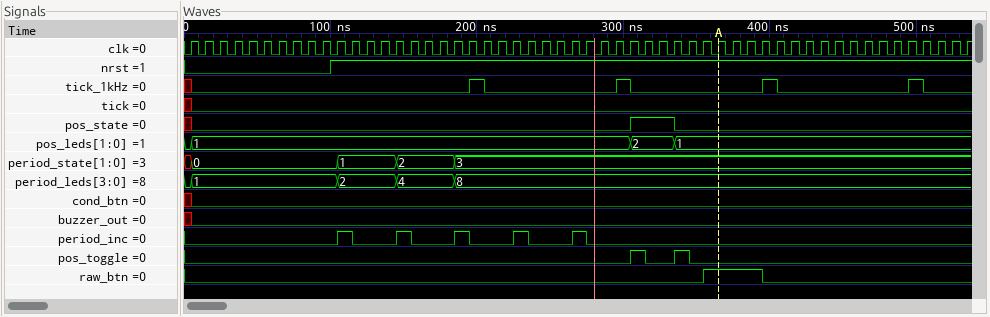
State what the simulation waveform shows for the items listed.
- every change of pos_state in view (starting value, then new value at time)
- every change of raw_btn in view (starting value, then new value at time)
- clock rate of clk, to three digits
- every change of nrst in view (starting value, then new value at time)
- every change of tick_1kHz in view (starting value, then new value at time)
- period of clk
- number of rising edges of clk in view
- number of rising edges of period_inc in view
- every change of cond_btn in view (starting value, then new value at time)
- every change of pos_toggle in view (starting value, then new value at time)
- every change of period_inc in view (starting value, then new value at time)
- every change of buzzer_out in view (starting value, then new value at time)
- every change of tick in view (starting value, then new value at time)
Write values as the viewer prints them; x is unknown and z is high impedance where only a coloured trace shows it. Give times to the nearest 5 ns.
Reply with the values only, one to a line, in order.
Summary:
x, 0 at 5 ns, 1 at 305 ns, 0 at 335 ns
0, 1 at 355 ns, 0 at 395 ns
100 MHz
0, 1 at 100 ns
x, 0 at 5 ns, 1 at 195 ns, 0 at 205 ns, 1 at 295 ns, 0 at 305 ns, 1 at 395 ns, 0 at 405 ns, 1 at 495 ns, 0 at 505 ns
10 ns
54
5
x, 0 at 5 ns
0, 1 at 305 ns, 0 at 315 ns, 1 at 335 ns, 0 at 345 ns
0, 1 at 105 ns, 0 at 115 ns, 1 at 145 ns, 0 at 155 ns, 1 at 185 ns, 0 at 195 ns, 1 at 225 ns, 0 at 235 ns, 1 at 265 ns, 0 at 275 ns
x, 0 at 5 ns
x, 0 at 5 ns
